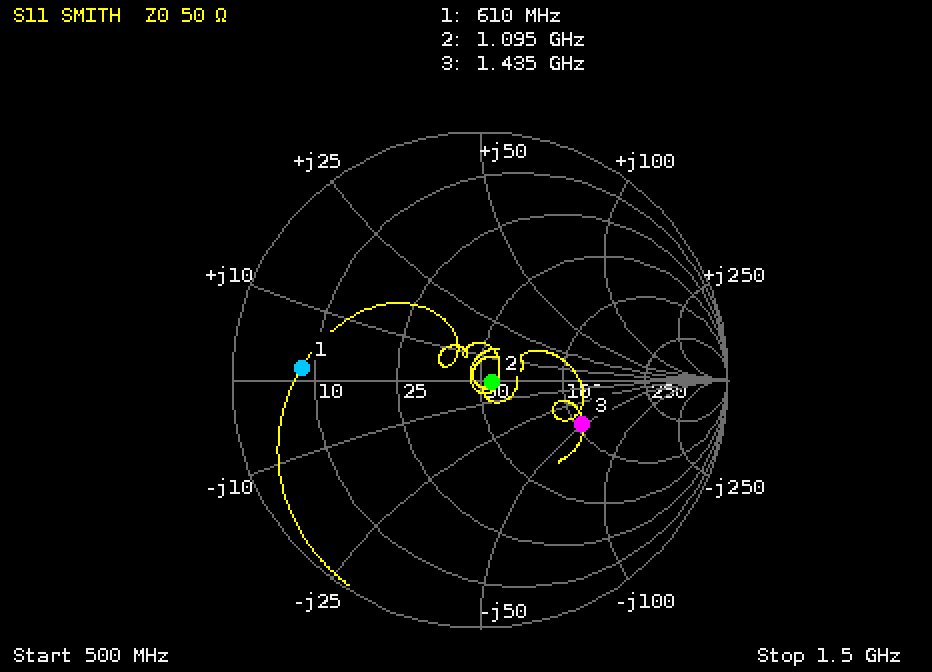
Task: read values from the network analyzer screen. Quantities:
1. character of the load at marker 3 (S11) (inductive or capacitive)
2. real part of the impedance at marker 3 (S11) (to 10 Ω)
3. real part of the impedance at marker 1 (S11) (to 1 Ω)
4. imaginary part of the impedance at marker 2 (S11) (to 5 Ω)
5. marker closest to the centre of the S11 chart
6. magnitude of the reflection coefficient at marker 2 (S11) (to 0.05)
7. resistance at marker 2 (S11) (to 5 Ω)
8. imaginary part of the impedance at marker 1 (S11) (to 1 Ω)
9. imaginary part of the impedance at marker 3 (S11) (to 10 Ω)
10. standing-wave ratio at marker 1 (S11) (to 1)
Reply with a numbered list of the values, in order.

1. capacitive
2. 110 Ω
3. 8 Ω
4. 0 Ω
5. marker 2
6. 0.05
7. 55 Ω
8. +2 Ω
9. -50 Ω
10. 6
